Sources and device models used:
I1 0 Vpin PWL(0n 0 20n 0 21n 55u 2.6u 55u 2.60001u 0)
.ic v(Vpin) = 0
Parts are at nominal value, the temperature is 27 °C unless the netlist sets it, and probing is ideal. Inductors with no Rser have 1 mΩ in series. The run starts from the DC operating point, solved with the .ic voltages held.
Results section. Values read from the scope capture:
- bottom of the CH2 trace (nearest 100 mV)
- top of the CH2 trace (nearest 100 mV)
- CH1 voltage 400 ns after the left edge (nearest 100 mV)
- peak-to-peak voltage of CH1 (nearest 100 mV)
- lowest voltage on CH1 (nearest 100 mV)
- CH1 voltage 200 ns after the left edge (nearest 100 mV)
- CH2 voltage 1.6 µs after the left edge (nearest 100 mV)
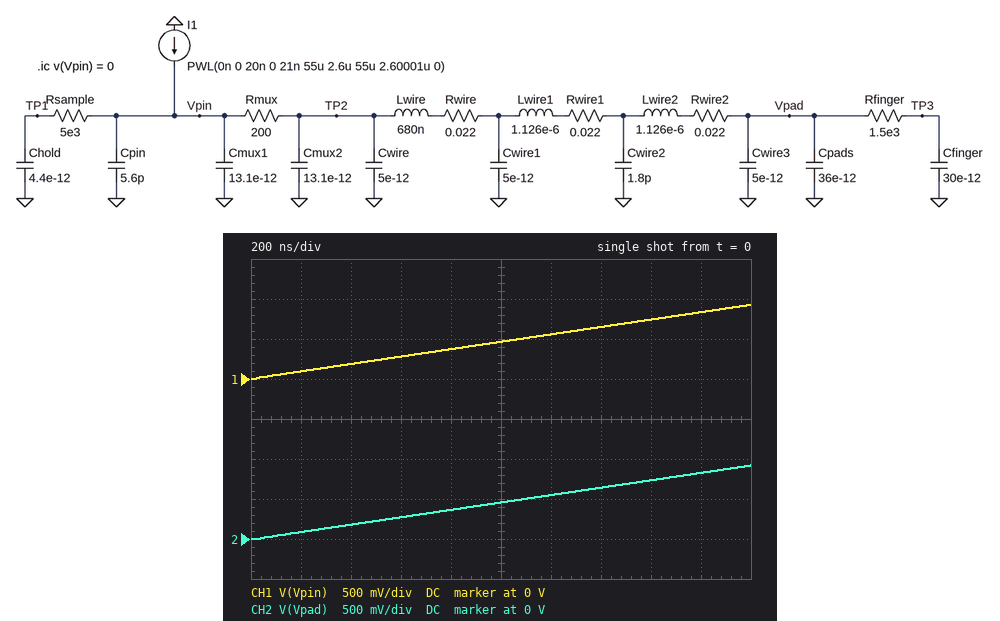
0 V
900 mV
200 mV
900 mV
0 V
100 mV
700 mV
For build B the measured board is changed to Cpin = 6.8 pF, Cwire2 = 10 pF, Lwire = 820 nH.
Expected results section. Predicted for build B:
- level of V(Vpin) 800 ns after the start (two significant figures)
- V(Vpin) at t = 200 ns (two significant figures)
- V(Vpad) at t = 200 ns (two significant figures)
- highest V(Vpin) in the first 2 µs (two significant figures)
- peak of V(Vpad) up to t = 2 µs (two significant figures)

350 mV
89 mV
80 mV
860 mV
850 mV
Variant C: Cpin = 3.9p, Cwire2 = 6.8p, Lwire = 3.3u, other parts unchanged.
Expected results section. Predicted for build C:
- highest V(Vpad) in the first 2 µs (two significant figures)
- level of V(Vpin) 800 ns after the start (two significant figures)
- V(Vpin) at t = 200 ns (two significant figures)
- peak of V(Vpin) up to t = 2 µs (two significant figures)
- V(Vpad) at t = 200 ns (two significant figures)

890 mV
360 mV
92 mV
900 mV
86 mV
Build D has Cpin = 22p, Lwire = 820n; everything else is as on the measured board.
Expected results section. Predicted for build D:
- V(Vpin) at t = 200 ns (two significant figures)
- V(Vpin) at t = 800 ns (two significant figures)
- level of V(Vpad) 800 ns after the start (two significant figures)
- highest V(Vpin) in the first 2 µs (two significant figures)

83 mV
330 mV
320 mV
810 mV
